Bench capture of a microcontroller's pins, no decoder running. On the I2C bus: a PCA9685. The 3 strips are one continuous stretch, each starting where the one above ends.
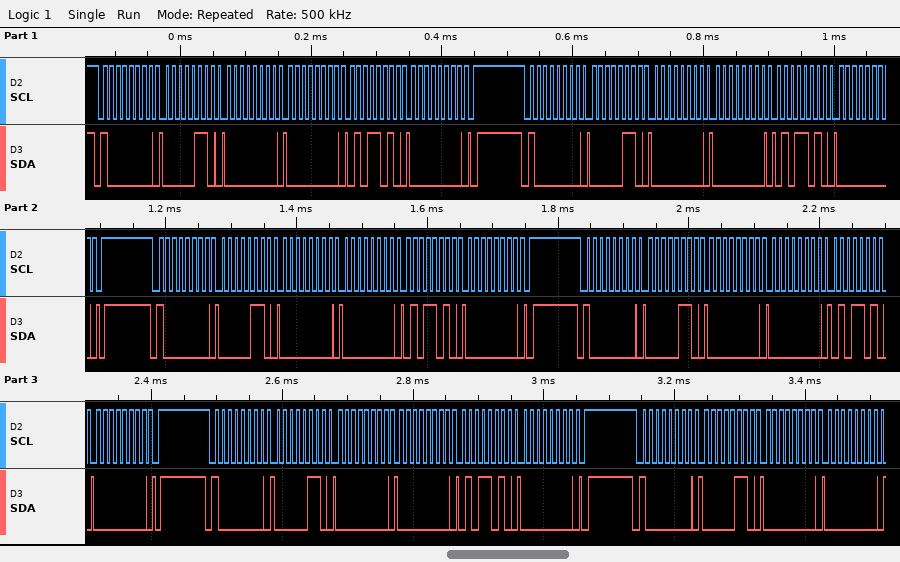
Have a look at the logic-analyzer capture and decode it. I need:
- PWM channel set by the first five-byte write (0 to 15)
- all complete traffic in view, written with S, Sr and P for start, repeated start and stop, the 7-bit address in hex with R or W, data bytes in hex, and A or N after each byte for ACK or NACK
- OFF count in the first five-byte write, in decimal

0
S 40W A 06 A 00 A 00 A 5A A 00 A P S 40W A 06 A 00 A 00 A 5A A 00 A P S 40W A 06 A 00 A 00 A 5A A 00 A P S 40W A 06 A 00 A 00 A 5A A 00 A P S 40W A 06 A 00 A 00 A 5A A 00 A P S 40W A 06 A 00 A 00 A
90
